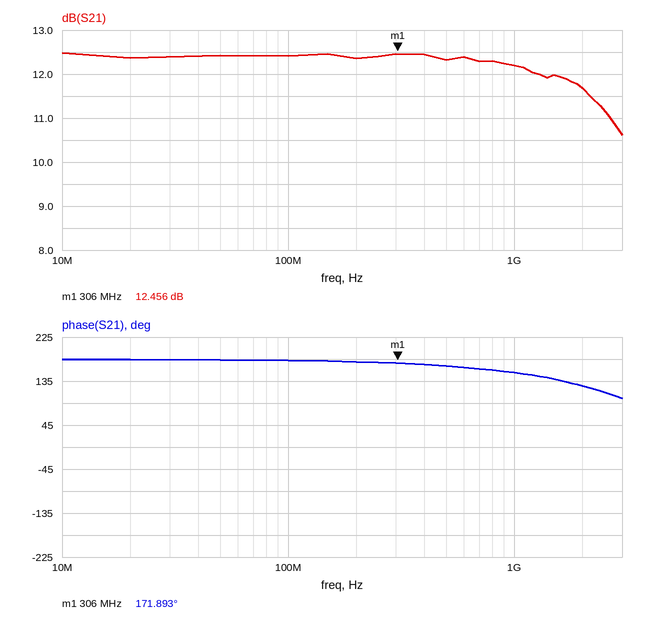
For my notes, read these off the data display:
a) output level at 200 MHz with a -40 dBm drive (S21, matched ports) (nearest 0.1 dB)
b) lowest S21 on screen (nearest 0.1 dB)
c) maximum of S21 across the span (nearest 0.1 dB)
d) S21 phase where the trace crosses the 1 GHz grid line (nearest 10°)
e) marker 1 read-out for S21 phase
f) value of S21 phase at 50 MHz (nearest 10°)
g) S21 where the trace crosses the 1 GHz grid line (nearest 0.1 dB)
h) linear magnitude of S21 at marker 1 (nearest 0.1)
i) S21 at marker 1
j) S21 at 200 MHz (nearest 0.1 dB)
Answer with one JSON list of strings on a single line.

["-27.6 dBm", "10.6 dB", "12.5 dB", "150°", "171.893°", "180°", "12.2 dB", "4.2", "12.456 dB", "12.4 dB"]
